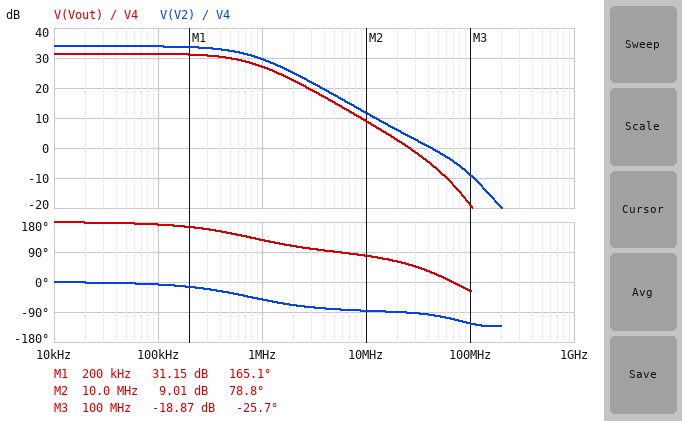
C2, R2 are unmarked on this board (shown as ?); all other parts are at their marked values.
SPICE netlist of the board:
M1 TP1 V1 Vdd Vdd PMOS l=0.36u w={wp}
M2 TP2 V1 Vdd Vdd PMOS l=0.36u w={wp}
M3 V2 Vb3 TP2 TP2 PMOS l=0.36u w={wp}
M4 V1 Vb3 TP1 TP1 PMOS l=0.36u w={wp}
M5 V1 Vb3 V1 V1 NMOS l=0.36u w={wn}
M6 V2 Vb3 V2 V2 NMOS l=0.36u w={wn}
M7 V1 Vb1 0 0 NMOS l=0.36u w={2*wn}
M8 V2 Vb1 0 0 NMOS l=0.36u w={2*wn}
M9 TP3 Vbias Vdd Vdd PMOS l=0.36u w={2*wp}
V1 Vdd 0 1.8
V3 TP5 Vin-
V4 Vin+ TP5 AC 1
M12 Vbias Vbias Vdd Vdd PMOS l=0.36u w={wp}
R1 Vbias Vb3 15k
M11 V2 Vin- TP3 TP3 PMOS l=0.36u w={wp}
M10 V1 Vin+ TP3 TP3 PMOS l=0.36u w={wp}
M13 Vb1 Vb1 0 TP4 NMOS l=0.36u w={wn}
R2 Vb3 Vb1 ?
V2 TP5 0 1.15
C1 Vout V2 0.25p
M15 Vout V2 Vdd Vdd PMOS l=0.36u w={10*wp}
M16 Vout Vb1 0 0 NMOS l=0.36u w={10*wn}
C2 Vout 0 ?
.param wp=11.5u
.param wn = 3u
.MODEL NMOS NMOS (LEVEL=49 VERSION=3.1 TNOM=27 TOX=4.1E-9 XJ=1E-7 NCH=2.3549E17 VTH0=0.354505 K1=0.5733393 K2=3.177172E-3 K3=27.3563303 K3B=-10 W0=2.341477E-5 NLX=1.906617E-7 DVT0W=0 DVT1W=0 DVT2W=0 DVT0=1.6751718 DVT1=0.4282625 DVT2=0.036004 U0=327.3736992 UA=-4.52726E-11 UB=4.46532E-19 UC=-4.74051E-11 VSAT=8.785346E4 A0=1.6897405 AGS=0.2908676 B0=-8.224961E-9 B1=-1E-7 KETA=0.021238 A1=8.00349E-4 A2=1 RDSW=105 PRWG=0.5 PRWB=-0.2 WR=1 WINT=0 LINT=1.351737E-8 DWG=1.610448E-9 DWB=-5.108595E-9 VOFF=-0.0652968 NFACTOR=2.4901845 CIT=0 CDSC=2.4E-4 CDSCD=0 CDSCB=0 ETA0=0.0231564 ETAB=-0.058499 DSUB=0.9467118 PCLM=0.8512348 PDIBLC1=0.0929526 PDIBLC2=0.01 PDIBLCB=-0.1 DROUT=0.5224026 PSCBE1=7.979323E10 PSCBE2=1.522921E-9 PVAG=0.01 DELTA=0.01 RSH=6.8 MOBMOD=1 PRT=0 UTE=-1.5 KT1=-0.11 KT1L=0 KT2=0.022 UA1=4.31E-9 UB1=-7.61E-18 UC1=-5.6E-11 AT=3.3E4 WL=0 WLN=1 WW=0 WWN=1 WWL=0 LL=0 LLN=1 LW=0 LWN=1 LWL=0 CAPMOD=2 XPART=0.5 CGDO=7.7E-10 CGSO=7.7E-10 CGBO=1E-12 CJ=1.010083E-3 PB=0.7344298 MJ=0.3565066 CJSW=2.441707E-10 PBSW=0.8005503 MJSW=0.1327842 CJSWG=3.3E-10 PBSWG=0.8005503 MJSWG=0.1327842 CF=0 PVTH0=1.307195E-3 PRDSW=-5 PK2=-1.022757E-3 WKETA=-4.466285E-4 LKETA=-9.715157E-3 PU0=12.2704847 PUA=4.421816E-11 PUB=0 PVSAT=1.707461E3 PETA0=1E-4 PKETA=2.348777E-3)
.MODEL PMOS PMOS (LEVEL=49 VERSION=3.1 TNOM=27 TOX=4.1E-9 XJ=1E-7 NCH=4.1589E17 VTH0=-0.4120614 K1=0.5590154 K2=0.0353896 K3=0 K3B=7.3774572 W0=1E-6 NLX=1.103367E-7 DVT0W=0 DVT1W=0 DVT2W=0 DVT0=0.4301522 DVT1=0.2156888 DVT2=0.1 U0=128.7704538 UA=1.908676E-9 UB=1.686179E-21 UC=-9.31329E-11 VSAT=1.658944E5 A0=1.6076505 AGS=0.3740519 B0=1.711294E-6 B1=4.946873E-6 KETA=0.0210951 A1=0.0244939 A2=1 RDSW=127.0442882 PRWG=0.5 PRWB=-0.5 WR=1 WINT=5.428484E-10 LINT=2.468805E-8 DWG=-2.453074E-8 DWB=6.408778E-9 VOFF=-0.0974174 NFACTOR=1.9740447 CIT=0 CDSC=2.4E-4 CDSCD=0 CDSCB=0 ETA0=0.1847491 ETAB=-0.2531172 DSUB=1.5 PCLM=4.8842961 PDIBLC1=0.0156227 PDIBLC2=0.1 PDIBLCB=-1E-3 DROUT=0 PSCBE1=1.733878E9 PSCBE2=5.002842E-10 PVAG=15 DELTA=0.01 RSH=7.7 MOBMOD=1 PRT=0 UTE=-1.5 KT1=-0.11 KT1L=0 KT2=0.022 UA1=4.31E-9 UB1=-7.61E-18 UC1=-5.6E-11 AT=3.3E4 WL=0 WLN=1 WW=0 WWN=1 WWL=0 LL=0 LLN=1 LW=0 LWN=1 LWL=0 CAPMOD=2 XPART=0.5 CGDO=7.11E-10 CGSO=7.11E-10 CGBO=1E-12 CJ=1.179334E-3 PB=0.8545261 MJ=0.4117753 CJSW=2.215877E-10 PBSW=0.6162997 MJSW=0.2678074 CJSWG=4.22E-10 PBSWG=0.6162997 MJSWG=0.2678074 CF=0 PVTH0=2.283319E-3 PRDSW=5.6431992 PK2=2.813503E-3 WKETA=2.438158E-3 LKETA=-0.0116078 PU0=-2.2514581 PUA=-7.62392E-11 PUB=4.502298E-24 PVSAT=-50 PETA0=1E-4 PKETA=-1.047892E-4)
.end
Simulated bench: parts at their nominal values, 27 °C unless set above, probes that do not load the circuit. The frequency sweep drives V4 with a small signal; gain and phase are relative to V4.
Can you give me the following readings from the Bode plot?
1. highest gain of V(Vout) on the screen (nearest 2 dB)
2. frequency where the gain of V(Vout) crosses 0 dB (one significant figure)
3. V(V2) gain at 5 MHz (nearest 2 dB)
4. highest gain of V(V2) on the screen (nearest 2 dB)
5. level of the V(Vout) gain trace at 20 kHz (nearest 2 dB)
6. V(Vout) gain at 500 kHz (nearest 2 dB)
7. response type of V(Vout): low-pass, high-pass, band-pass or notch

32 dB
30 MHz
18 dB
34 dB
32 dB
30 dB
low-pass
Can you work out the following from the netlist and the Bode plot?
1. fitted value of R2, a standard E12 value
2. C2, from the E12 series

12 kΩ
3.3 pF
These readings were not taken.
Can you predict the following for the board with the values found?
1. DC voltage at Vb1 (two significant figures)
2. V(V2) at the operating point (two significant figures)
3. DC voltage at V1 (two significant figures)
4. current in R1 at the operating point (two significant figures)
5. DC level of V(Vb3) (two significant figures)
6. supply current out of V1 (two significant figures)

570 mV
1.3 V
1.3 V
23 µA
850 mV
98 µA
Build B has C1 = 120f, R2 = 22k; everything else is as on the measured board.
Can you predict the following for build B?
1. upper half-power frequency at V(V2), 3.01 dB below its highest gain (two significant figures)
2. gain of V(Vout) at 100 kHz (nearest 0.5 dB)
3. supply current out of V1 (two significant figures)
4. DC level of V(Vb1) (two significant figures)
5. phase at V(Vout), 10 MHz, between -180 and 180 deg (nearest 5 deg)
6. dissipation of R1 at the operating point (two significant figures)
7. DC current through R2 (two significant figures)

1.2 MHz
14.0 dB
51 µA
550 mV
65 deg
4.7 µW
18 µA
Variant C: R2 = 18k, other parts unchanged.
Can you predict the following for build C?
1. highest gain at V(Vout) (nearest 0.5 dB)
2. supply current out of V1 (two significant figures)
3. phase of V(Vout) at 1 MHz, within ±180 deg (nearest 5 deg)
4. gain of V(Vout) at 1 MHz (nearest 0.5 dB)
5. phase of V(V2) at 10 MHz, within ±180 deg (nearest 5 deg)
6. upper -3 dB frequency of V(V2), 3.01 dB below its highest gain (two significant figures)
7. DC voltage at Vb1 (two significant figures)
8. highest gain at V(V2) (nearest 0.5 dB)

23.0 dB
65 µA
130 deg
19.5 dB
-90 deg
870 kHz
560 mV
34.0 dB
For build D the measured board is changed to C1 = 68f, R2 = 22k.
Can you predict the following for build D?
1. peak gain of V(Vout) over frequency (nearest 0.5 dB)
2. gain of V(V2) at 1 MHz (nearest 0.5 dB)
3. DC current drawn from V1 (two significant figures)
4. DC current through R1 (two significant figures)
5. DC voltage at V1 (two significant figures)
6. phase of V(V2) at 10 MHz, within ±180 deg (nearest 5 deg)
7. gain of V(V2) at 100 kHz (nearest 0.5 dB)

14.0 dB
32.0 dB
51 µA
18 µA
1.4 V
-95 deg
33.5 dB
